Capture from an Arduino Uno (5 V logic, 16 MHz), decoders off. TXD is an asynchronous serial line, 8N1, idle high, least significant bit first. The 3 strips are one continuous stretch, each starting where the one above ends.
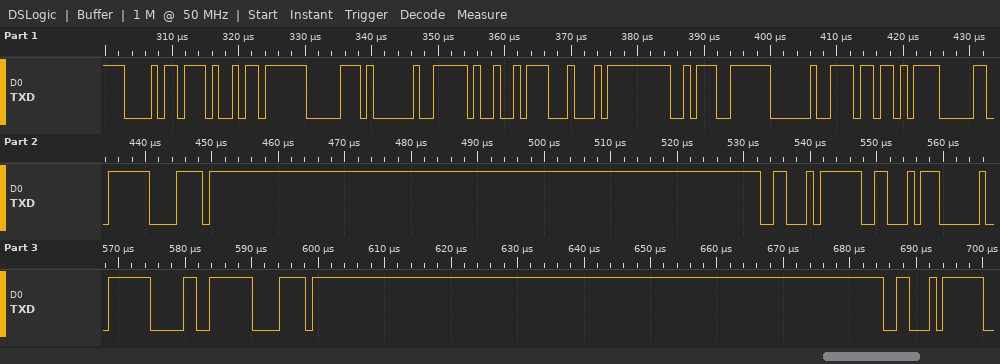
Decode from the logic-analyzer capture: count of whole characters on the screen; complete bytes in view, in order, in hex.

17
68 69 70 20 49 44 3A 20 5B 30 78 46 46 20 30 78 46
